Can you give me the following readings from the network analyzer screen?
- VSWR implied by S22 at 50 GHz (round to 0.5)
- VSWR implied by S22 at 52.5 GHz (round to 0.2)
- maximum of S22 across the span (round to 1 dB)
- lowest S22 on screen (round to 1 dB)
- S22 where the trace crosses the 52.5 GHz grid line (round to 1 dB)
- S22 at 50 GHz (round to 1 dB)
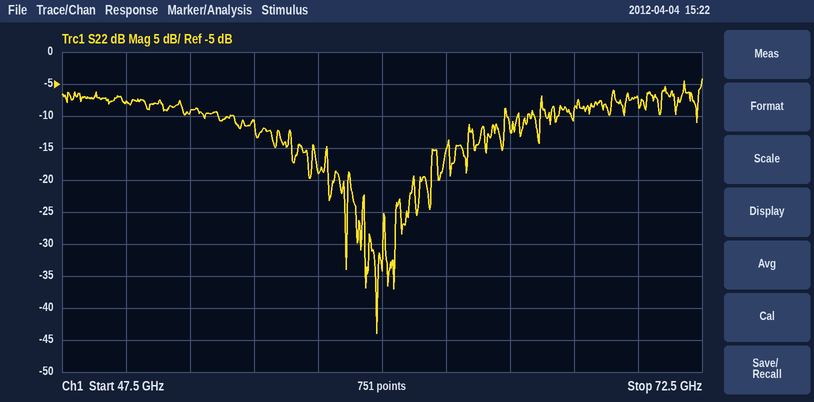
2.5
2.0
-4 dB
-44 dB
-9 dB
-8 dB
